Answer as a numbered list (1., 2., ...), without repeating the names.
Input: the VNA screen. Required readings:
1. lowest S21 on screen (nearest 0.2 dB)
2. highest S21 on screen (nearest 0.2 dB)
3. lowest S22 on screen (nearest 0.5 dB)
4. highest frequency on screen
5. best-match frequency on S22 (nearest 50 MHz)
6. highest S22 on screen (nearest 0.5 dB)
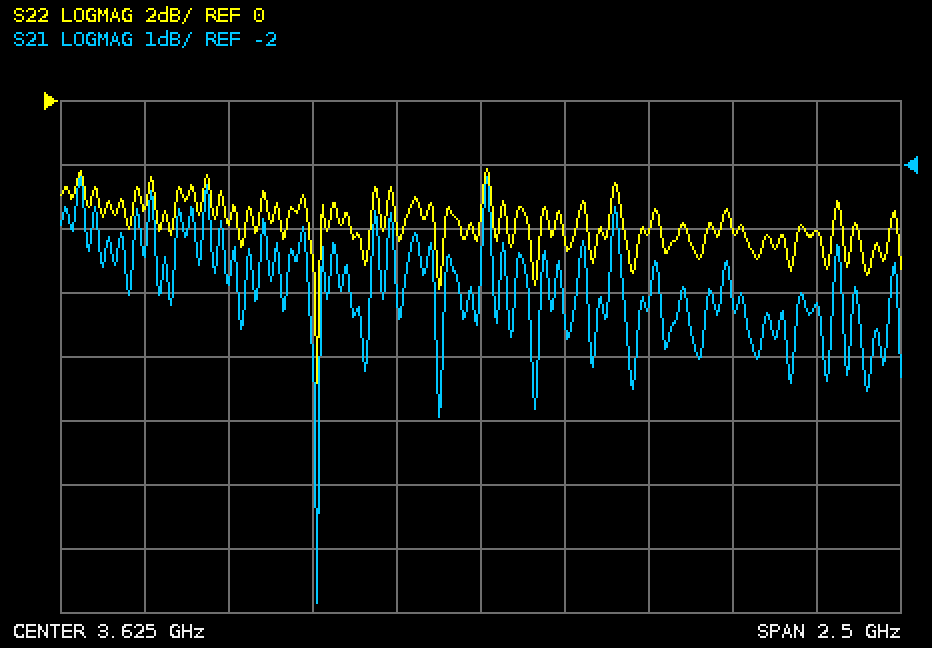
1. -8.8 dB
2. -2.2 dB
3. -9.0 dB
4. 4.875 GHz
5. 3.15 GHz
6. -2.0 dB
